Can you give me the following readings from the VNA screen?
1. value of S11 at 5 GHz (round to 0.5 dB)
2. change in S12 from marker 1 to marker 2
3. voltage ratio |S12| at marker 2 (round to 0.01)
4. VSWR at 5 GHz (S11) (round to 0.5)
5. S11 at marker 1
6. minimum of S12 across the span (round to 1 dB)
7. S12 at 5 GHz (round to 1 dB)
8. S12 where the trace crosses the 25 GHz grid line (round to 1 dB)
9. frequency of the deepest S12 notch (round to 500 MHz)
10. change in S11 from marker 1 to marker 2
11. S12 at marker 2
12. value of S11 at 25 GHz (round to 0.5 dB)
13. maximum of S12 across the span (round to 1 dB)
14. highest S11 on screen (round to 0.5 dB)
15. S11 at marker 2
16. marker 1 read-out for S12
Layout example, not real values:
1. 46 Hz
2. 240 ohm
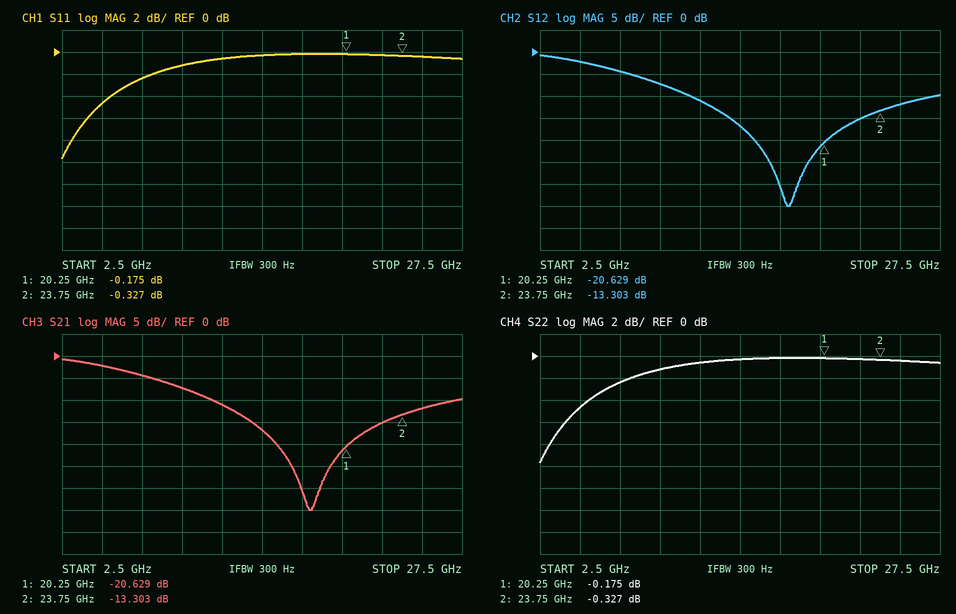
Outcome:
1. -4.5 dB
2. 7.326 dB
3. 0.22
4. 4.0
5. -0.175 dB
6. -35 dB
7. -2 dB
8. -12 dB
9. 18.0 GHz
10. -0.152 dB
11. -13.303 dB
12. -0.5 dB
13. -1 dB
14. 0.0 dB
15. -0.327 dB
16. -20.629 dB
